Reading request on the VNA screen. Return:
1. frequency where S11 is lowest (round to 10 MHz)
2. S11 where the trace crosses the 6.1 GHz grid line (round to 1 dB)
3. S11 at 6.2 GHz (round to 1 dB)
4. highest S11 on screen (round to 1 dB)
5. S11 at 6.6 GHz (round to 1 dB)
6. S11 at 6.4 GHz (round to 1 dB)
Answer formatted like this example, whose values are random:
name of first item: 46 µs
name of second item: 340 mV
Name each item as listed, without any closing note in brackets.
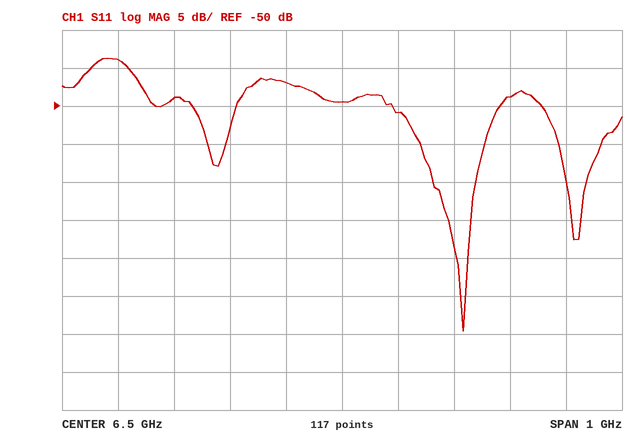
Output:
frequency where S11 is lowest: 6.72 GHz
S11 where the trace crosses the 6.1 GHz grid line: -44 dB
S11 at 6.2 GHz: -49 dB
highest S11 on screen: -44 dB
S11 at 6.6 GHz: -51 dB
S11 at 6.4 GHz: -47 dB
